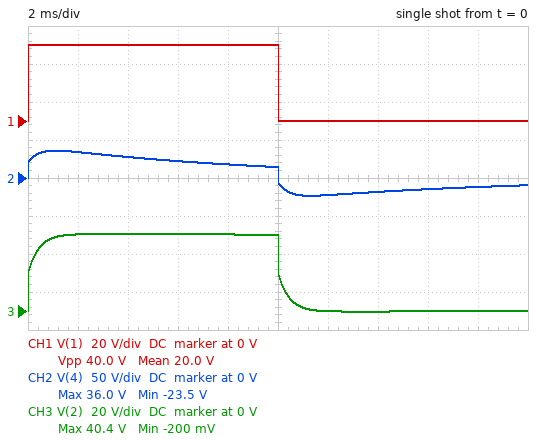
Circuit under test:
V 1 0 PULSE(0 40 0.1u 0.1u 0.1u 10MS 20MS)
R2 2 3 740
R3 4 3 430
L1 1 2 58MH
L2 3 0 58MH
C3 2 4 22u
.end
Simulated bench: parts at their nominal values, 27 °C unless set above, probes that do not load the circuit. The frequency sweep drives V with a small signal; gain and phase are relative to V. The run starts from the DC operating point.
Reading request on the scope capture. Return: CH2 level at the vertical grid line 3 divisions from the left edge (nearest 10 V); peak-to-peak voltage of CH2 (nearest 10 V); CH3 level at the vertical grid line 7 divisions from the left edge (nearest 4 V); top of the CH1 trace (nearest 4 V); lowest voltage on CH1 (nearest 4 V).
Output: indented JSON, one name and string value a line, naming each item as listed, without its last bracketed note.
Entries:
{
  "CH2 level at the vertical grid line 3 divisions from the left edge": "20 V",
  "peak-to-peak voltage of CH2": "60 V",
  "CH3 level at the vertical grid line 7 divisions from the left edge": "0 V",
  "top of the CH1 trace": "40 V",
  "lowest voltage on CH1": "0 V"
}
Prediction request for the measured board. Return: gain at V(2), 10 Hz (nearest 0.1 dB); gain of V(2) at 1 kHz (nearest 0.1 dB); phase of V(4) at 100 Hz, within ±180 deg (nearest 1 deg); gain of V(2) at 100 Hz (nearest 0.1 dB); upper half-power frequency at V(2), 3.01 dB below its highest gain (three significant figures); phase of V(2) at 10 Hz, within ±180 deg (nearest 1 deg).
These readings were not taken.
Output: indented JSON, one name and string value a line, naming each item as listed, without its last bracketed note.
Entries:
{
  "gain at V(2), 10 Hz": "0 dB",
  "gain of V(2) at 1 kHz": "-4.7 dB",
  "phase of V(4) at 100 Hz, within ±180 deg": "2 deg",
  "gain of V(2) at 100 Hz": "-0.1 dB",
  "upper half-power frequency at V(2), 3.01 dB below its highest gain": "514 Hz",
  "phase of V(2) at 10 Hz, within ±180 deg": "0 deg"
}
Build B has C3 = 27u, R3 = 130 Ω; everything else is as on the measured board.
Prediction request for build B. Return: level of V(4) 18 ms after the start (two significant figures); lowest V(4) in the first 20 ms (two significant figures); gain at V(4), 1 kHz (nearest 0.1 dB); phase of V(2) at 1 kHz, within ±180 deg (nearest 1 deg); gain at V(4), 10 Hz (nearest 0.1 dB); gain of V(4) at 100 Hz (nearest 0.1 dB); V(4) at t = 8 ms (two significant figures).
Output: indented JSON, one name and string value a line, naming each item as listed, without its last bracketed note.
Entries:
{
  "level of V(4) 18 ms after the start": "-3.4 V",
  "lowest V(4) in the first 20 ms": "-29 V",
  "gain at V(4), 1 kHz": "-5.7 dB",
  "phase of V(2) at 1 kHz, within ±180 deg": "-8 deg",
  "gain at V(4), 10 Hz": "-13.0 dB",
  "gain of V(4) at 100 Hz": "0.1 dB",
  "V(4) at t = 8 ms": "3.4 V"
}
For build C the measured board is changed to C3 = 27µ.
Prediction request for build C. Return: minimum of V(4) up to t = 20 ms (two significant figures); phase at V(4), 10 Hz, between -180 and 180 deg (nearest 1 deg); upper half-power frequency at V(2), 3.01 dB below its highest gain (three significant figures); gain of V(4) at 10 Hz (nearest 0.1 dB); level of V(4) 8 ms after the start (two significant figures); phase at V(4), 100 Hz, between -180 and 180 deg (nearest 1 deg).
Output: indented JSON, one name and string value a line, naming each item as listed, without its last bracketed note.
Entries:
{
  "minimum of V(4) up to t = 20 ms": "-21 V",
  "phase at V(4), 10 Hz, between -180 and 180 deg": "54 deg",
  "upper half-power frequency at V(2), 3.01 dB below its highest gain": "516 Hz",
  "gain of V(4) at 10 Hz": "-4.5 dB",
  "level of V(4) 8 ms after the start": "21 V",
  "phase at V(4), 100 Hz, between -180 and 180 deg": "0 deg"
}
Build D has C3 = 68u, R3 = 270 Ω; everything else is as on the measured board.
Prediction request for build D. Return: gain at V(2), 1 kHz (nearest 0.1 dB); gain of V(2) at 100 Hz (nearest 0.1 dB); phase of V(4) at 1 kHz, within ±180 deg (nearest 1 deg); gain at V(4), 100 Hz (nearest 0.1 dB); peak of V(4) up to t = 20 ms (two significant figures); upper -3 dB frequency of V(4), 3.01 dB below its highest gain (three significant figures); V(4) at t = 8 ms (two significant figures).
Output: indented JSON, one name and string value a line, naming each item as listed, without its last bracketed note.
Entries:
{
  "gain at V(2), 1 kHz": "-5.2 dB",
  "gain of V(2) at 100 Hz": "-0.3 dB",
  "phase of V(4) at 1 kHz, within ±180 deg": "-13 deg",
  "gain at V(4), 100 Hz": "-0.2 dB",
  "peak of V(4) up to t = 20 ms": "37 V",
  "upper -3 dB frequency of V(4), 3.01 dB below its highest gain": "396 Hz",
  "V(4) at t = 8 ms": "27 V"
}
